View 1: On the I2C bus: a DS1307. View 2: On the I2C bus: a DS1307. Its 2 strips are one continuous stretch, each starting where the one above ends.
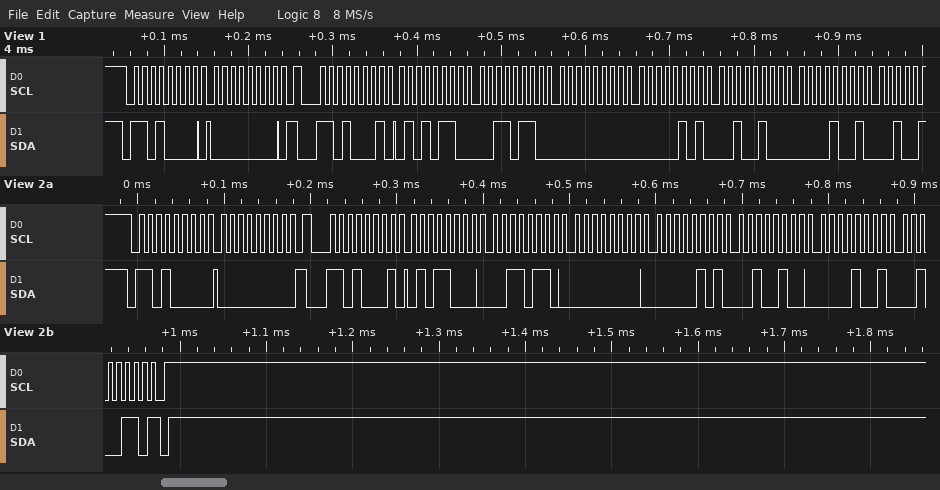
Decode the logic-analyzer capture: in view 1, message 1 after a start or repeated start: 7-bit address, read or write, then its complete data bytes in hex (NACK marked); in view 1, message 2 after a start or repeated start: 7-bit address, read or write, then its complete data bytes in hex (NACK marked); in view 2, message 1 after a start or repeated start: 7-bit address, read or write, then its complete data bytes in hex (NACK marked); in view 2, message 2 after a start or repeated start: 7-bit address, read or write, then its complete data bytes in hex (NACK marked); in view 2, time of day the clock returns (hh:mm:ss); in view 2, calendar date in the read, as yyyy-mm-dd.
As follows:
0x68 write: 00
0x68 read: 56 36 00 05 24 09
0x68 write: 00
0x68 read: 58 36 00 05 24 09 26 NACK
00:36:58
2026-09-24
